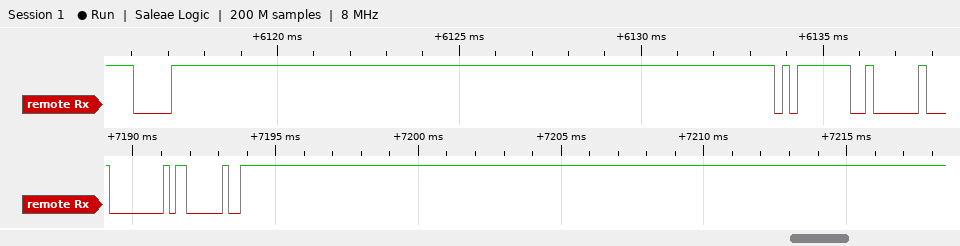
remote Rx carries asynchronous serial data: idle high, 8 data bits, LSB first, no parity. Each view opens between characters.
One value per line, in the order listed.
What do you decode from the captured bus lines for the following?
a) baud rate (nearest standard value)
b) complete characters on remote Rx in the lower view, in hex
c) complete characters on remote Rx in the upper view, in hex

4800 baud
00, 03, FE
F0, FD, 02
